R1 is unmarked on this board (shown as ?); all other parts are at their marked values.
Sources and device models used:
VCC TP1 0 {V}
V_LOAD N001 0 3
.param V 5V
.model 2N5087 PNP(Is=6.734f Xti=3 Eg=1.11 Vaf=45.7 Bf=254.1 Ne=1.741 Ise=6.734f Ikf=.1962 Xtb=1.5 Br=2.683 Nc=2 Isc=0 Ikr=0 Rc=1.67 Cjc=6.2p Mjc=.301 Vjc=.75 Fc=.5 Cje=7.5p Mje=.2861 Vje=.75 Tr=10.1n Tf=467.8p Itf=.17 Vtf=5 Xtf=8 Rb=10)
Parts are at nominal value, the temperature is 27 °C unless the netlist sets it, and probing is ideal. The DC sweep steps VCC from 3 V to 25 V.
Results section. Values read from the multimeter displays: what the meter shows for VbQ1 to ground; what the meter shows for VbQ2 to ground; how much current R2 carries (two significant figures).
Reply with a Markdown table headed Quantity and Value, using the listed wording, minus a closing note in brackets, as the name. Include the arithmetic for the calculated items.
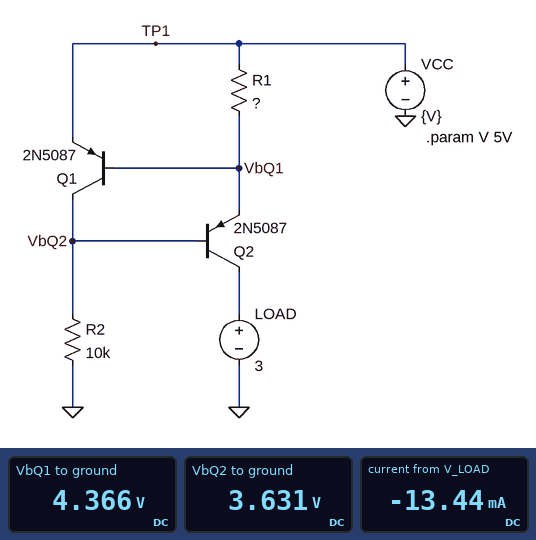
| Quantity | Value |
|---|---|
| what the meter shows for VbQ1 to ground | 4.366 V |
| what the meter shows for VbQ2 to ground | 3.631 V |
| how much current R2 carries | (3.631 V) / 10 kΩ = 360 µA |
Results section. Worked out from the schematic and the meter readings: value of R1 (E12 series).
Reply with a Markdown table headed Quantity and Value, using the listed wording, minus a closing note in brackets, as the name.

| Quantity | Value |
|---|---|
| value of R1 | 47 Ω |
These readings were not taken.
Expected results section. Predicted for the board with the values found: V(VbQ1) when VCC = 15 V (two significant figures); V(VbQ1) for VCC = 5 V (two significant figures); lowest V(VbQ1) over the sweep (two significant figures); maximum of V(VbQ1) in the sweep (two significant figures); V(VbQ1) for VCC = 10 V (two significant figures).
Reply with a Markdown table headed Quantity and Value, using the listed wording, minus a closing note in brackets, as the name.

| Quantity | Value |
|---|---|
| V(VbQ1) when VCC = 15 V | 14 V |
| V(VbQ1) for VCC = 5 V | 4.4 V |
| lowest V(VbQ1) over the sweep | 3.0 V |
| maximum of V(VbQ1) in the sweep | 24 V |
| V(VbQ1) for VCC = 10 V | 9.3 V |
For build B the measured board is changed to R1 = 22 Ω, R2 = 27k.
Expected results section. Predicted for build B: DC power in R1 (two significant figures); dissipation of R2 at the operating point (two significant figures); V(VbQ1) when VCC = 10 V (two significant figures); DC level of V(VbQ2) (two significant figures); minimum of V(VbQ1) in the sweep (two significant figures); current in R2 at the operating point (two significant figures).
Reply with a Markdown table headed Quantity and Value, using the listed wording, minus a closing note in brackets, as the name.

| Quantity | Value |
|---|---|
| DC power in R1 | 15 mW |
| dissipation of R2 at the operating point | 500 µW |
| V(VbQ1) when VCC = 10 V | 9.4 V |
| DC level of V(VbQ2) | 3.7 V |
| minimum of V(VbQ1) in the sweep | 3.0 V |
| current in R2 at the operating point | 140 µA |
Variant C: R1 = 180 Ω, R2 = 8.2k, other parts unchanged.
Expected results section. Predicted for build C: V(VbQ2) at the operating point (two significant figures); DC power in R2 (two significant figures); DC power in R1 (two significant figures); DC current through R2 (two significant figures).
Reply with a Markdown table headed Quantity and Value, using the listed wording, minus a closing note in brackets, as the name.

| Quantity | Value |
|---|---|
| V(VbQ2) at the operating point | 3.7 V |
| DC power in R2 | 1.6 mW |
| DC power in R1 | 2.3 mW |
| DC current through R2 | 450 µA |
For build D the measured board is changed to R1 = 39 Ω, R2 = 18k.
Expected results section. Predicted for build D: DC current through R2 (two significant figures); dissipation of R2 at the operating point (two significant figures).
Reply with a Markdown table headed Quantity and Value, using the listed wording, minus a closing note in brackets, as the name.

| Quantity | Value |
|---|---|
| DC current through R2 | 200 µA |
| dissipation of R2 at the operating point | 740 µW |
